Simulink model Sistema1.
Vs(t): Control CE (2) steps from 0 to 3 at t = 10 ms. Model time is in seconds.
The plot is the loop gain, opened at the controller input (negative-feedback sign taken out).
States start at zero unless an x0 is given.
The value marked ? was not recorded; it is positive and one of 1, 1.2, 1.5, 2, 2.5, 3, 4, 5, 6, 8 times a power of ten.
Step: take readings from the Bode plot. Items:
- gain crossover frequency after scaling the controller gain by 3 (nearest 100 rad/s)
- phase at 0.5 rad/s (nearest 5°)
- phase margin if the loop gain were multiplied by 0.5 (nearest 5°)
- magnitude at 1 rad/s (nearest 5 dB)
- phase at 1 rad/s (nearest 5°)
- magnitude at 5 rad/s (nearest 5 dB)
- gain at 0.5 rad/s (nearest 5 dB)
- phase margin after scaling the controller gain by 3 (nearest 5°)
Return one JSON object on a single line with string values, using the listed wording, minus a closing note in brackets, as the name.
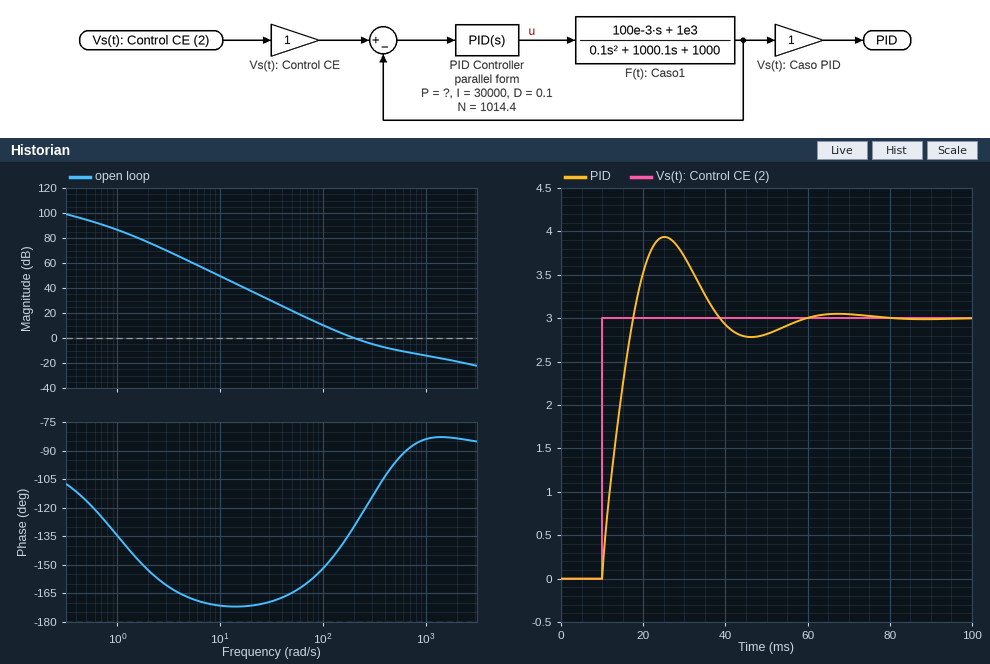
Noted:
{"gain crossover frequency after scaling the controller gain by 3": "500 rad/s", "phase at 0.5 rad/s": "-115°", "phase margin if the loop gain were multiplied by 0.5": "35°", "magnitude at 1 rad/s": "85 dB", "phase at 1 rad/s": "-135°", "magnitude at 5 rad/s": "60 dB", "gain at 0.5 rad/s": "95 dB", "phase margin after scaling the controller gain by 3": "85°"}
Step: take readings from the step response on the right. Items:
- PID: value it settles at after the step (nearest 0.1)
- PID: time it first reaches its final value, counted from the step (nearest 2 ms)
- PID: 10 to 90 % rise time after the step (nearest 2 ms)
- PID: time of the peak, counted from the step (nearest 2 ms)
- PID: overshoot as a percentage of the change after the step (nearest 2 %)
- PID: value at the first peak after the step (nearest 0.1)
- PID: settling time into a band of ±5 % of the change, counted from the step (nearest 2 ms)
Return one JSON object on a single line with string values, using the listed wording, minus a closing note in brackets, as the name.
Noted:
{"PID: value it settles at after the step": "3.0", "PID: time it first reaches its final value, counted from the step": "8 ms", "PID: 10 to 90 % rise time after the step": "6 ms", "PID: time of the peak, counted from the step": "16 ms", "PID: overshoot as a percentage of the change after the step": "32 %", "PID: value at the first peak after the step": "3.9", "PID: settling time into a band of ±5 % of the change, counted from the step": "42 ms"}
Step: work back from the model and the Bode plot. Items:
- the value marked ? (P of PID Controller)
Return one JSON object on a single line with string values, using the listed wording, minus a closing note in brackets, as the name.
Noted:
{"the value marked ?": "150"}
